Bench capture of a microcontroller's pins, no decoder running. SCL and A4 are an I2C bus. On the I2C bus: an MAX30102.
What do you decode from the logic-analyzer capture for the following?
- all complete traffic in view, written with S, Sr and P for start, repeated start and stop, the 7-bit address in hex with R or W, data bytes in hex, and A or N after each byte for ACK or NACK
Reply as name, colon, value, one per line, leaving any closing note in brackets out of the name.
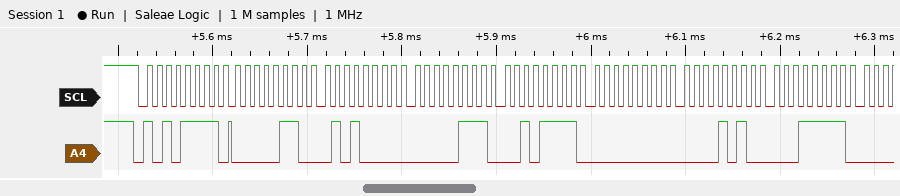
all complete traffic in view, written with S, Sr and P for start, repeated start and stop, the 7-bit address in hex with R or W, data bytes in hex, and A or N after each byte for ACK or NACK: S 57R A 06 A 50 A 07 A 2F A 00 A 0A A 1F A
